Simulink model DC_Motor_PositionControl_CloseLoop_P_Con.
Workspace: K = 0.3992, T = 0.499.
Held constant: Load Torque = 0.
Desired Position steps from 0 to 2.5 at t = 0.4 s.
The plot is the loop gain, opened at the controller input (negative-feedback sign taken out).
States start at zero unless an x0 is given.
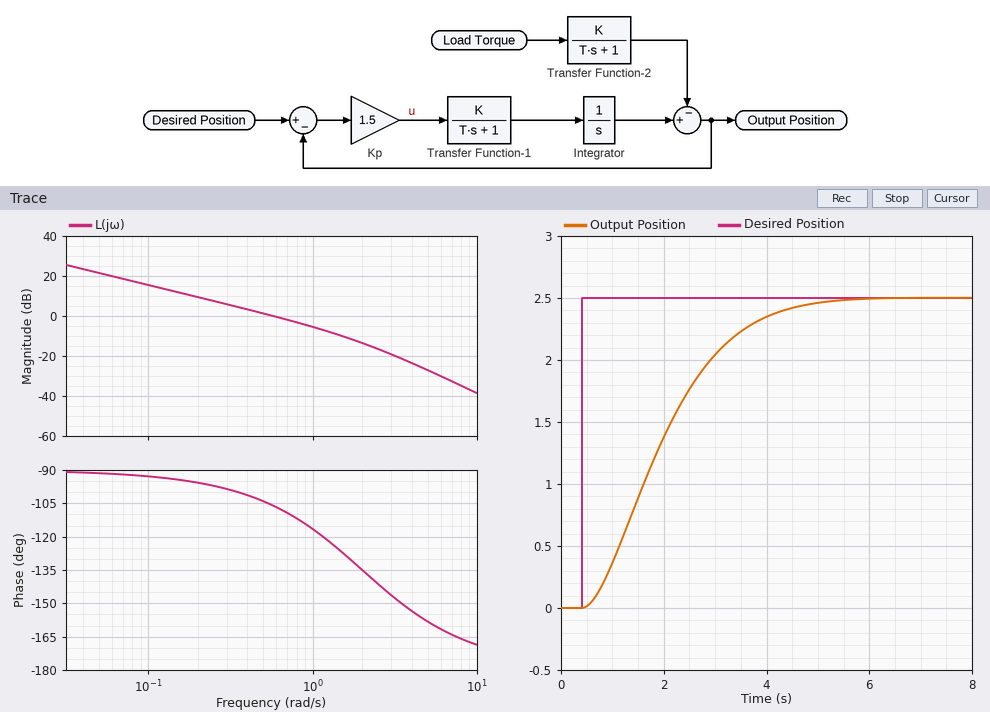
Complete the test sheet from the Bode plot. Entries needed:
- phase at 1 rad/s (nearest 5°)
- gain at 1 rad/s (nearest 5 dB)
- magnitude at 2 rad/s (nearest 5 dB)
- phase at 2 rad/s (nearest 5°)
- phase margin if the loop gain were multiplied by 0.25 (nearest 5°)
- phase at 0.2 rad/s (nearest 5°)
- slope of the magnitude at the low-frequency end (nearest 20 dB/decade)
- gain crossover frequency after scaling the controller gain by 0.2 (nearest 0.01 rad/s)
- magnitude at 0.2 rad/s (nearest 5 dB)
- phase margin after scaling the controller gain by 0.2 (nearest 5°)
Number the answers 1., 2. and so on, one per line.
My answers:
1. -115°
2. -5 dB
3. -15 dB
4. -135°
5. 85°
6. -95°
7. -20 dB/decade
8. 0.12 rad/s
9. 10 dB
10. 85°
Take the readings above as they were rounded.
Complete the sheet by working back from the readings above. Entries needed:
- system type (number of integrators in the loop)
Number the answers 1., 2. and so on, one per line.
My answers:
1. 1
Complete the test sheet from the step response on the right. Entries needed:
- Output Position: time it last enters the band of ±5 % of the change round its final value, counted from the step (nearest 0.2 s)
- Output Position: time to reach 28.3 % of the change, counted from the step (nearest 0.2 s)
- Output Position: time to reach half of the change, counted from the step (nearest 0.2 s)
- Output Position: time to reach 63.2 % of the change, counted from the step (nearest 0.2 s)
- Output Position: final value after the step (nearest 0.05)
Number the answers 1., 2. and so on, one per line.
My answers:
1. 3.8 s
2. 1.0 s
3. 1.4 s
4. 1.8 s
5. 2.50
